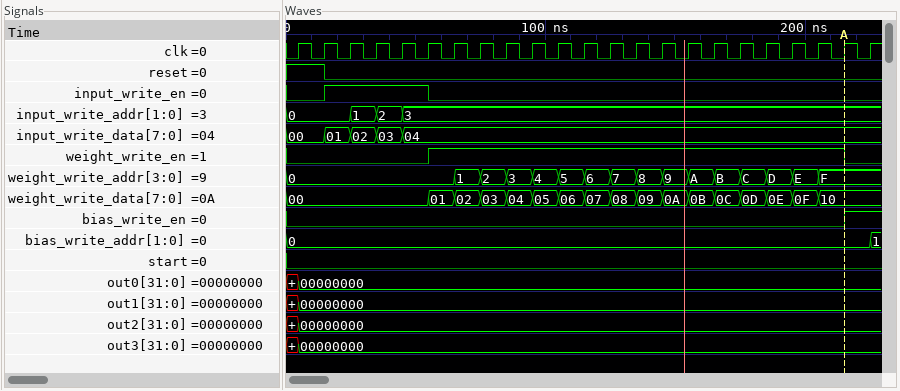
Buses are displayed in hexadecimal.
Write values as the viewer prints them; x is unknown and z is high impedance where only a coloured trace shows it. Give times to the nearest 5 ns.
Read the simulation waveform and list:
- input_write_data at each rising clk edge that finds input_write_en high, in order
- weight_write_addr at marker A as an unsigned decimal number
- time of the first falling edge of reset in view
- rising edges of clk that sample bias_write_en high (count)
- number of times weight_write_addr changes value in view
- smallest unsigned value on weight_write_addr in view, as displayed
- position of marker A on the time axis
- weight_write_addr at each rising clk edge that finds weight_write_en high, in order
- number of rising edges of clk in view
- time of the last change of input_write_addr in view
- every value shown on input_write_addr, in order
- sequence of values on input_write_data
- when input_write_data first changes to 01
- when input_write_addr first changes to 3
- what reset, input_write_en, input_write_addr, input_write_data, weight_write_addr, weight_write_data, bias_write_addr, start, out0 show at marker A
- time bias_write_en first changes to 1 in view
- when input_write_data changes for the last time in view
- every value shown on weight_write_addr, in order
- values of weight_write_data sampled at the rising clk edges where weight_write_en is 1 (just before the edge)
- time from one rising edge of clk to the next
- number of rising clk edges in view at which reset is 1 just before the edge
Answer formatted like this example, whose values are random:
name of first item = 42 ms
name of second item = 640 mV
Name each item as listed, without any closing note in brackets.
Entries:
input_write_data at each rising clk edge that finds input_write_en high, in order = 01, 02, 03, 04
weight_write_addr at marker A as an unsigned decimal number = 15
time of the first falling edge of reset in view = 15 ns
rising edges of clk that sample bias_write_en high = 1
number of times weight_write_addr changes value in view = 15
smallest unsigned value on weight_write_addr in view, as displayed = 0
position of marker A on the time axis = 215 ns
weight_write_addr at each rising clk edge that finds weight_write_en high, in order = 0, 1, 2, 3, 4, 5, 6, 7, 8, 9, A, B, C, D, E, F
number of rising edges of clk in view = 23
time of the last change of input_write_addr in view = 45 ns
every value shown on input_write_addr, in order = 0, 1, 2, 3
sequence of values on input_write_data = 00, 01, 02, 03, 04
when input_write_data first changes to 01 = 15 ns
when input_write_addr first changes to 3 = 45 ns
what reset, input_write_en, input_write_addr, input_write_data, weight_write_addr, weight_write_data, bias_write_addr, start, out0 show at marker A = reset=0, input_write_en=0, input_write_addr=3, input_write_data=04, weight_write_addr=F, weight_write_data=10, bias_write_addr=0, start=0, out0=00000000
time bias_write_en first changes to 1 in view = 215 ns
when input_write_data changes for the last time in view = 45 ns
every value shown on weight_write_addr, in order = 0, 1, 2, 3, 4, 5, 6, 7, 8, 9, A, B, C, D, E, F
values of weight_write_data sampled at the rising clk edges where weight_write_en is 1 = 01, 02, 03, 04, 05, 06, 07, 08, 09, 0A, 0B, 0C, 0D, 0E, 0F, 10
time from one rising edge of clk to the next = 10 ns
number of rising clk edges in view at which reset is 1 just before the edge = 2
